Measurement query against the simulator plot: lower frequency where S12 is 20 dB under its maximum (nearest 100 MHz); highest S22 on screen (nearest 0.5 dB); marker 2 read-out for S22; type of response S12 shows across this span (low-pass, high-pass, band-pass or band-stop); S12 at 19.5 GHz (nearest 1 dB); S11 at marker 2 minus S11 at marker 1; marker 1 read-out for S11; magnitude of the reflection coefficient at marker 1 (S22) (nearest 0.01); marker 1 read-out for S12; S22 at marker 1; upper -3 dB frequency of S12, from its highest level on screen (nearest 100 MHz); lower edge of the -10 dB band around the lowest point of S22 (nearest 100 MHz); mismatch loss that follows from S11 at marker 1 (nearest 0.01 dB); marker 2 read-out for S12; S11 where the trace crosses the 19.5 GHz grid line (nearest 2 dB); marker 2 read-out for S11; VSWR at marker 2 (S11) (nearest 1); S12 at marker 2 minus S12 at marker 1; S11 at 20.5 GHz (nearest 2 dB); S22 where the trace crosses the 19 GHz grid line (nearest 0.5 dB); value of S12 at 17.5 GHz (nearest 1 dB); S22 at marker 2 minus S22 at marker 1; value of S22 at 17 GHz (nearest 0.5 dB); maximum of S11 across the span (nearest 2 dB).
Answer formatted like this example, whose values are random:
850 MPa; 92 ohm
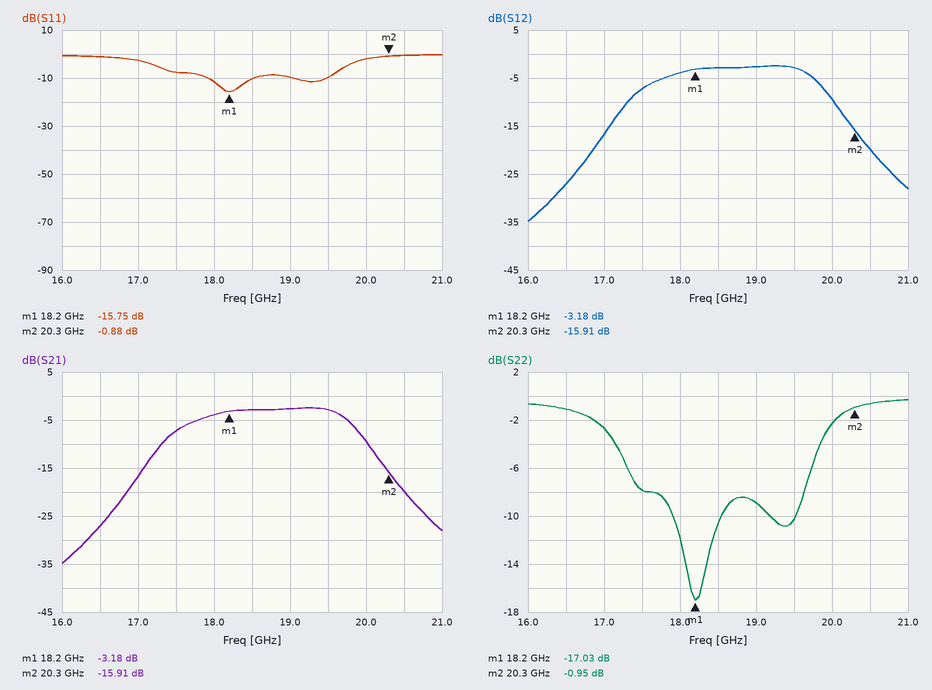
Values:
16.7 GHz; -0.5 dB; -0.95 dB; band-pass; -3 dB; 14.87 dB; -15.75 dB; 0.14; -3.18 dB; -17.03 dB; 19.8 GHz; 17.9 GHz; 0.12 dB; -15.91 dB; -10 dB; -0.88 dB; 20; -12.73 dB; 0 dB; -9.0 dB; -7 dB; 16.08 dB; -2.5 dB; 0 dB
